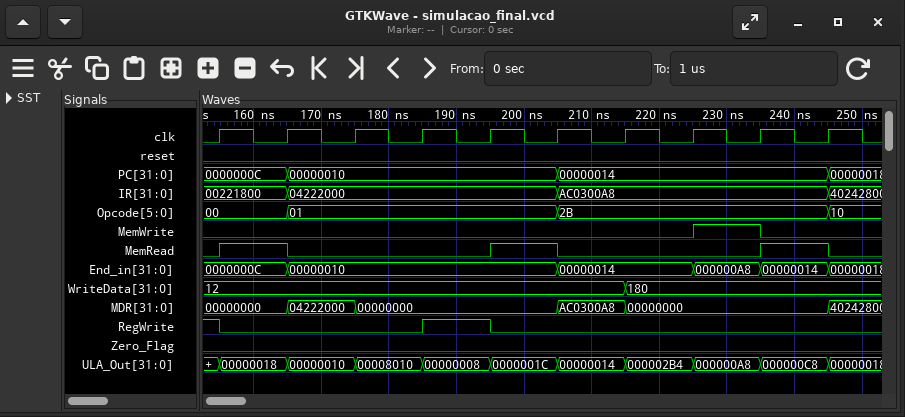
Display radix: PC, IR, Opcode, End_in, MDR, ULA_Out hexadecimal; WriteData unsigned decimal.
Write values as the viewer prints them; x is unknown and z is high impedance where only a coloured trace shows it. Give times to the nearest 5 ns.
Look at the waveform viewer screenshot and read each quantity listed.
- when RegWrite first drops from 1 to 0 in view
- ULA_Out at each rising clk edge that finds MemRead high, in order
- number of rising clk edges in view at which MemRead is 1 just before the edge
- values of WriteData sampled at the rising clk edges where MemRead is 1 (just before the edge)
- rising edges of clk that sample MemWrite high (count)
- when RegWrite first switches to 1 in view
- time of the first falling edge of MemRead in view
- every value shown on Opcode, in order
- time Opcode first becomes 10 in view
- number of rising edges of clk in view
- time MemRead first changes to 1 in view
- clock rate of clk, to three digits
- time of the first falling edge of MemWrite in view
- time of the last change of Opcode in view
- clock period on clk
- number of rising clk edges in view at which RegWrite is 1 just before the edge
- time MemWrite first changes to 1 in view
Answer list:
155 ns
00000018, 0000001C, 000000C8
3
12, 12, 180
1
185 ns
165 ns
00, 01, 2B, 10
245 ns
10
155 ns
100 MHz
235 ns
245 ns
10 ns
2
225 ns
